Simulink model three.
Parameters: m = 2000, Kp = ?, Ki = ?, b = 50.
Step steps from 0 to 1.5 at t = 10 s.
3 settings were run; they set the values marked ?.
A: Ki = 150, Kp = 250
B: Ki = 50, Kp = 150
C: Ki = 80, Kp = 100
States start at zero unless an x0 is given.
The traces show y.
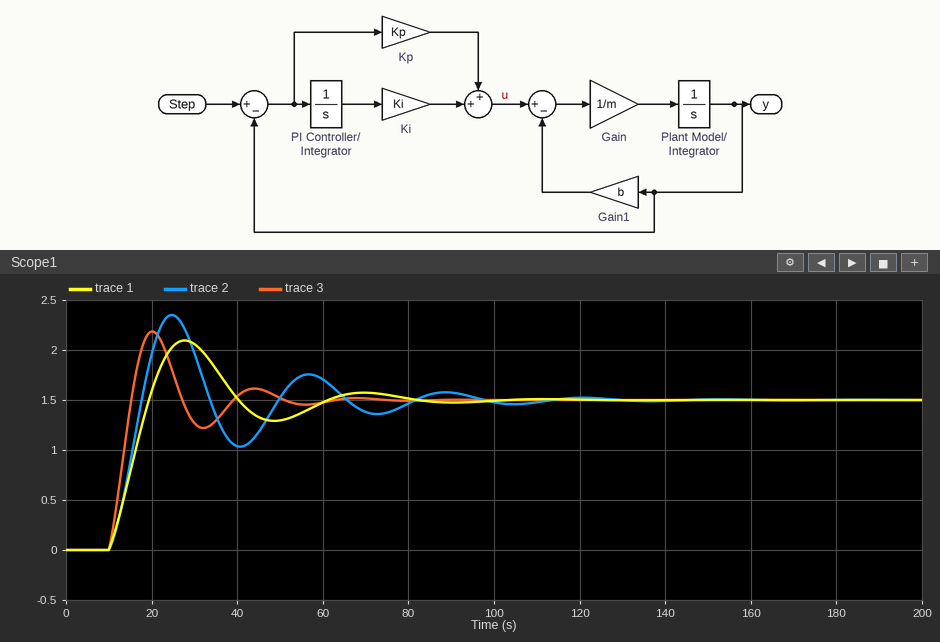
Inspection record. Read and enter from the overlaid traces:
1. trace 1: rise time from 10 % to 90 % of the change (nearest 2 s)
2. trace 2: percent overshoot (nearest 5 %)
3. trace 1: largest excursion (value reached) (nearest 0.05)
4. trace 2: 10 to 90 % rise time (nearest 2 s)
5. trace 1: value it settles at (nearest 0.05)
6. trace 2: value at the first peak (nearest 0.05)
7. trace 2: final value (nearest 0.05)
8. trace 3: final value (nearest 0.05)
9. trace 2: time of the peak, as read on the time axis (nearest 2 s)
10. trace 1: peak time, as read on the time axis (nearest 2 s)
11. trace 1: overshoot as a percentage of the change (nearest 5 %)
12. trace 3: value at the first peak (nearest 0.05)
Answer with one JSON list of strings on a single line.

["8 s", "55 %", "2.10", "6 s", "1.50", "2.35", "1.50", "1.50", "24 s", "28 s", "40 %", "2.20"]
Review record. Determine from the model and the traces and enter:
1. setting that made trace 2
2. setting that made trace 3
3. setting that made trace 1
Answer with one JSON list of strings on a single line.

["C", "A", "B"]
